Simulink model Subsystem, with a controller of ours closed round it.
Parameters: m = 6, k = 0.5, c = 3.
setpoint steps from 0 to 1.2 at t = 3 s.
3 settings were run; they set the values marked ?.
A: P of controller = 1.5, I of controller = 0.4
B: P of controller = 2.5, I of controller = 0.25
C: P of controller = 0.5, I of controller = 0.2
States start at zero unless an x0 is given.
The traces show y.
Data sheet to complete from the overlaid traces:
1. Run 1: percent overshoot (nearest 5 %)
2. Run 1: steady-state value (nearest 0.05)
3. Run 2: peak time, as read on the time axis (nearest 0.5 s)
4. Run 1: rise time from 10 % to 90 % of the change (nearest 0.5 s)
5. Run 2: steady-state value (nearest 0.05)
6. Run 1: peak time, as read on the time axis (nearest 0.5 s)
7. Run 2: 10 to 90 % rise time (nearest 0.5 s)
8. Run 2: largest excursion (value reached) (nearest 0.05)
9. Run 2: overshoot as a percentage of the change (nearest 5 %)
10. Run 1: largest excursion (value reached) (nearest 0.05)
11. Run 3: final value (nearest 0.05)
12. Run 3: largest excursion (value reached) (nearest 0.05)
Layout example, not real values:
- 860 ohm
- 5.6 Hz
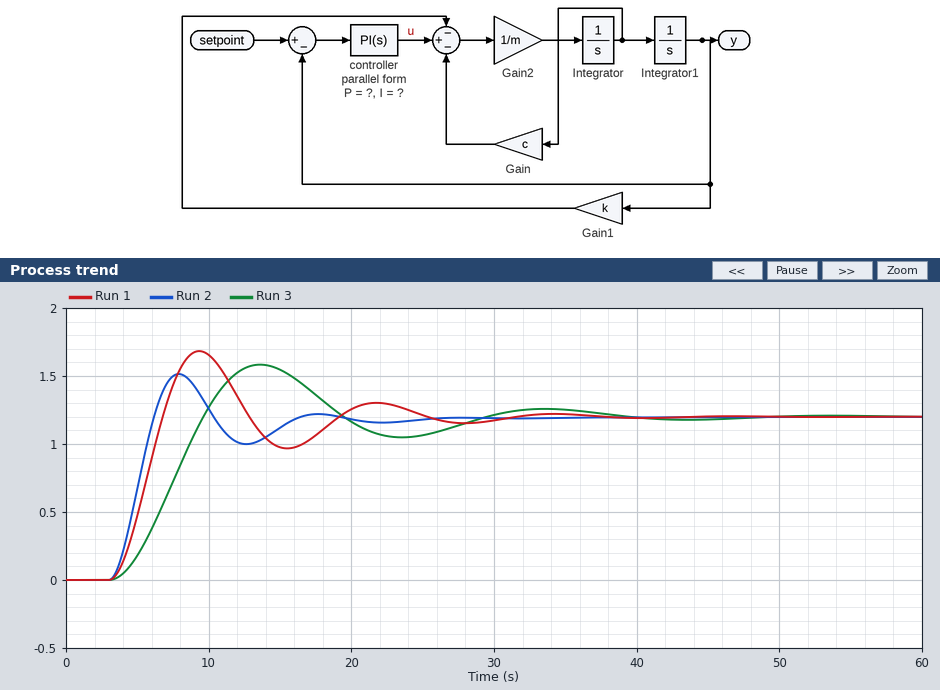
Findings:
- 40 %
- 1.20
- 8.0 s
- 2.5 s
- 1.20
- 9.5 s
- 2.0 s
- 1.50
- 25 %
- 1.70
- 1.20
- 1.60
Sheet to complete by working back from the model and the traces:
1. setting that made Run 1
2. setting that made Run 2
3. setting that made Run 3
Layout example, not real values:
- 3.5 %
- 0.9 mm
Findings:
- A
- B
- C
